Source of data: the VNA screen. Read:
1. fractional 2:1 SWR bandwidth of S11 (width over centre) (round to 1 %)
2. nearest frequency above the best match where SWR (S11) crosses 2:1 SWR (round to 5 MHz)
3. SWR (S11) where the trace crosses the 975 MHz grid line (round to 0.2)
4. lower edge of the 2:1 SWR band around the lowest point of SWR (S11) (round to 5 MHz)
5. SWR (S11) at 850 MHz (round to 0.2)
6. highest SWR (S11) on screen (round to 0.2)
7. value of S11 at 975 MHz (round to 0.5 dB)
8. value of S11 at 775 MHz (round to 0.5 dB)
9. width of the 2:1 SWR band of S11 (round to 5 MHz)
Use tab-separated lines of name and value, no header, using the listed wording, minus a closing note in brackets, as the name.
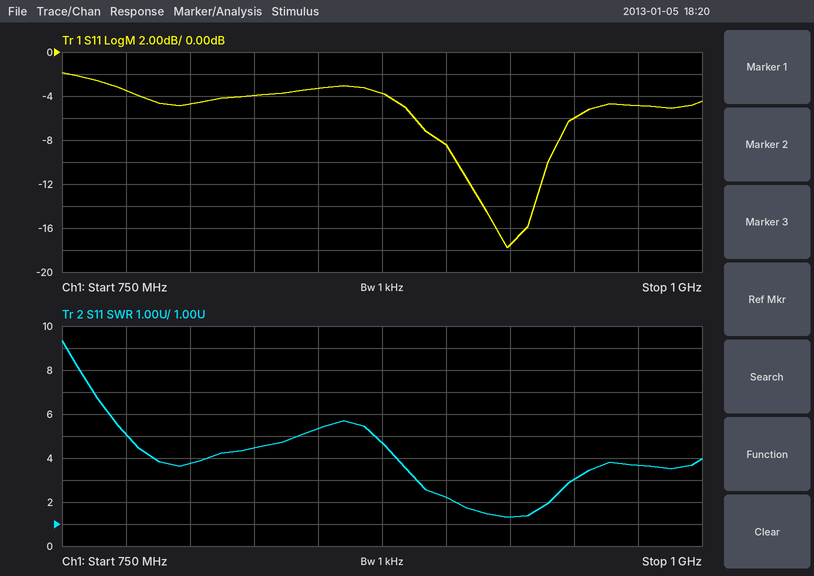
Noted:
fractional 2:1 SWR bandwidth of S11 (width over centre)	4 %
nearest frequency above the best match where SWR (S11) crosses 2:1 SWR	940 MHz
SWR (S11) where the trace crosses the 975 MHz grid line	3.6
lower edge of the 2:1 SWR band around the lowest point of SWR (S11)	905 MHz
SWR (S11) at 850 MHz	5.4
highest SWR (S11) on screen	9.4
value of S11 at 975 MHz	-5.0 dB
value of S11 at 775 MHz	-3.5 dB
width of the 2:1 SWR band of S11	35 MHz
